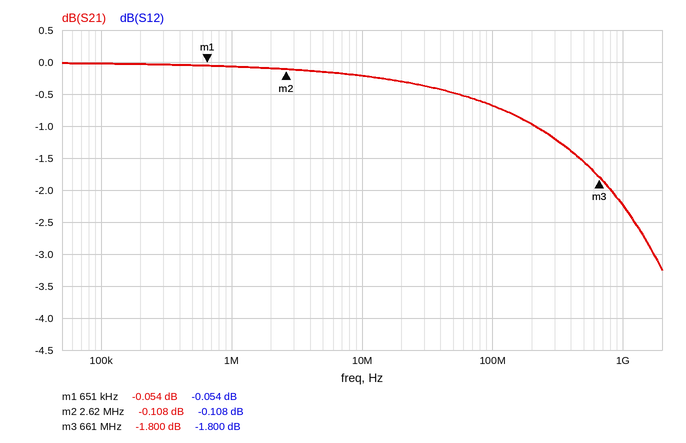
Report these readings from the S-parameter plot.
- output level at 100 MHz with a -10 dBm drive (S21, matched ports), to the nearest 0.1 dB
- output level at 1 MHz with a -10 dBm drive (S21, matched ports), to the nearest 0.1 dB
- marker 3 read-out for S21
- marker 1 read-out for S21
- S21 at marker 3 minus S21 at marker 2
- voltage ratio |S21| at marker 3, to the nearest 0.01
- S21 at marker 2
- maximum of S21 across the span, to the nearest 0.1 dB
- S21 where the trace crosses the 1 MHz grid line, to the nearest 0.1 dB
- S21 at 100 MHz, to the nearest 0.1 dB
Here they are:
-10.7 dBm
-10.1 dBm
-1.800 dB
-0.054 dB
-1.692 dB
0.81
-0.108 dB
0.0 dB
-0.1 dB
-0.7 dB
